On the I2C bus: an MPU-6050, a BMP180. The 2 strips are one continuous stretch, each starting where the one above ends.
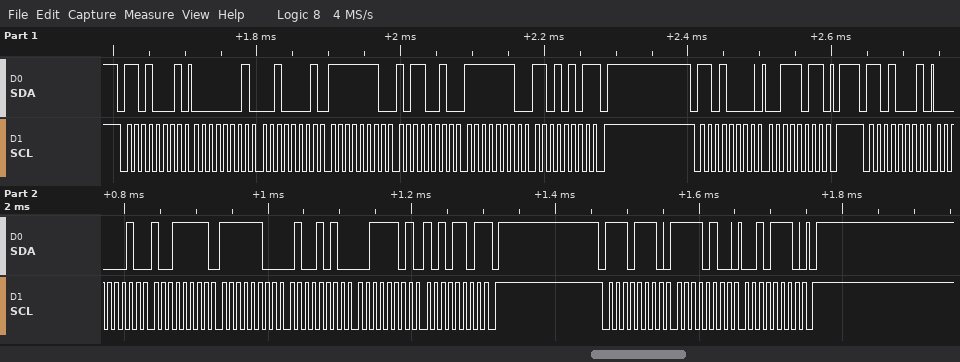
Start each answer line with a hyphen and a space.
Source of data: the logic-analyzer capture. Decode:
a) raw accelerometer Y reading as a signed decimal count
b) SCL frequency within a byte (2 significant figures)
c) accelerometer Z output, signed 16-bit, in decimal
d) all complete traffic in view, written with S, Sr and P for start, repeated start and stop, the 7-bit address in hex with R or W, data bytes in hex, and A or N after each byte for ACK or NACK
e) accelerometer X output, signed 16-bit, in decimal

- -950
- 100 kHz
- 15789
- S 68R A 01 A 21 A FE A B2 A FE A D5 N P S 68W A 3B A P S 68R A 02 A 9F A FC A 4A A 3D A AD N P S 77W A F4 A 2E A P
- 671
